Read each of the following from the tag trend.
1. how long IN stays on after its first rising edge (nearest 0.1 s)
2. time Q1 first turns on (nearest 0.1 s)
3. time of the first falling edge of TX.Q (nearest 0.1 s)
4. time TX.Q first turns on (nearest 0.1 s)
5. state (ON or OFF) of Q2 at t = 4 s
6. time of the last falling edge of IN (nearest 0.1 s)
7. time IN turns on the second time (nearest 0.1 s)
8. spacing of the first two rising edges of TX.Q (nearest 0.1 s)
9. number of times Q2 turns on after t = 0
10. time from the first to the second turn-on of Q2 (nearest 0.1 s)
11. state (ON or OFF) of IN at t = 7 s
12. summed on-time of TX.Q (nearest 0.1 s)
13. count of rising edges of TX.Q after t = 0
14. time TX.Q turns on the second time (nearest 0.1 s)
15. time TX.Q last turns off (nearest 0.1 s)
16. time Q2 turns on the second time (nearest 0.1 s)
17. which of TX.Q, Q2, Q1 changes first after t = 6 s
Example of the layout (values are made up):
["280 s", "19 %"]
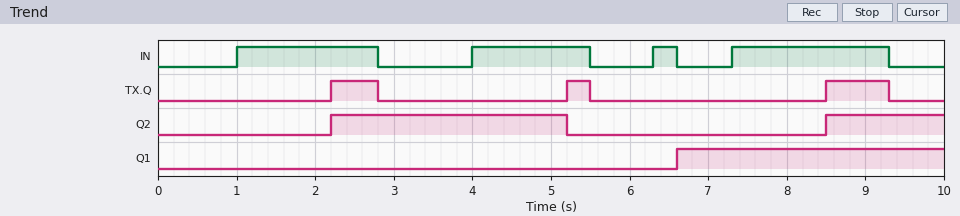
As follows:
["1.8 s", "6.6 s", "2.8 s", "2.2 s", "ON", "9.3 s", "4.0 s", "3.0 s", "2", "6.3 s", "OFF", "1.7 s", "3", "5.2 s", "9.3 s", "8.5 s", "Q1"]
